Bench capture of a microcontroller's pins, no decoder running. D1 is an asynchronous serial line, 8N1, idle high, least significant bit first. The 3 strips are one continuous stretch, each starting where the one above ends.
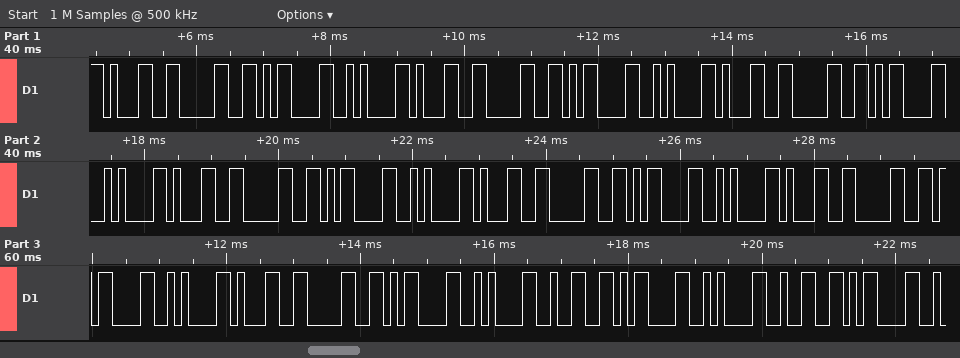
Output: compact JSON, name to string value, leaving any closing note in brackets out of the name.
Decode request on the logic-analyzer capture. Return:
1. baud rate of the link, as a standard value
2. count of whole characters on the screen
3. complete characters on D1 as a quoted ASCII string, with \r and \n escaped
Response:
{"baud rate of the link, as a standard value": "9600 baud", "count of whole characters on the screen": "33", "complete characters on D1 as a quoted ASCII string, with \\r and \\n escaped": "\"10\\r\\n10\\r\\n10\\r\\n10\\r\\n10\\r\\n10\\r\\n10\\r\\n2\\r\\n2\\r\""}
